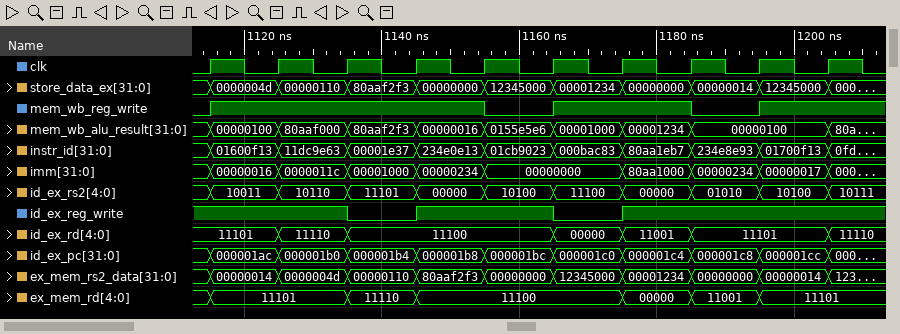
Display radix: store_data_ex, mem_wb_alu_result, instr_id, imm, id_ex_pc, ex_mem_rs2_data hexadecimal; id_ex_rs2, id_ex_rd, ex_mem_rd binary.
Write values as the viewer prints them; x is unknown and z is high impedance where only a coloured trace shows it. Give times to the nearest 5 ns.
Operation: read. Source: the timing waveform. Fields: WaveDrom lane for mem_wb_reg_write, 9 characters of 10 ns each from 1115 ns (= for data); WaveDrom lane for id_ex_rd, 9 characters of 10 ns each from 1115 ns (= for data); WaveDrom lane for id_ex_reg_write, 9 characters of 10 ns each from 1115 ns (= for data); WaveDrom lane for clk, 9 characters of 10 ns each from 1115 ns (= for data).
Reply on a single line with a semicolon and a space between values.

{name: 'mem_wb_reg_write', wave: '1...01.01'}; {name: 'id_ex_rd', wave: '===..===.', data: '11101 11110 11100 00000 11001 11101'}; {name: 'id_ex_reg_write', wave: '1.01.01..'}; {name: 'clk', wave: 'p........'}
